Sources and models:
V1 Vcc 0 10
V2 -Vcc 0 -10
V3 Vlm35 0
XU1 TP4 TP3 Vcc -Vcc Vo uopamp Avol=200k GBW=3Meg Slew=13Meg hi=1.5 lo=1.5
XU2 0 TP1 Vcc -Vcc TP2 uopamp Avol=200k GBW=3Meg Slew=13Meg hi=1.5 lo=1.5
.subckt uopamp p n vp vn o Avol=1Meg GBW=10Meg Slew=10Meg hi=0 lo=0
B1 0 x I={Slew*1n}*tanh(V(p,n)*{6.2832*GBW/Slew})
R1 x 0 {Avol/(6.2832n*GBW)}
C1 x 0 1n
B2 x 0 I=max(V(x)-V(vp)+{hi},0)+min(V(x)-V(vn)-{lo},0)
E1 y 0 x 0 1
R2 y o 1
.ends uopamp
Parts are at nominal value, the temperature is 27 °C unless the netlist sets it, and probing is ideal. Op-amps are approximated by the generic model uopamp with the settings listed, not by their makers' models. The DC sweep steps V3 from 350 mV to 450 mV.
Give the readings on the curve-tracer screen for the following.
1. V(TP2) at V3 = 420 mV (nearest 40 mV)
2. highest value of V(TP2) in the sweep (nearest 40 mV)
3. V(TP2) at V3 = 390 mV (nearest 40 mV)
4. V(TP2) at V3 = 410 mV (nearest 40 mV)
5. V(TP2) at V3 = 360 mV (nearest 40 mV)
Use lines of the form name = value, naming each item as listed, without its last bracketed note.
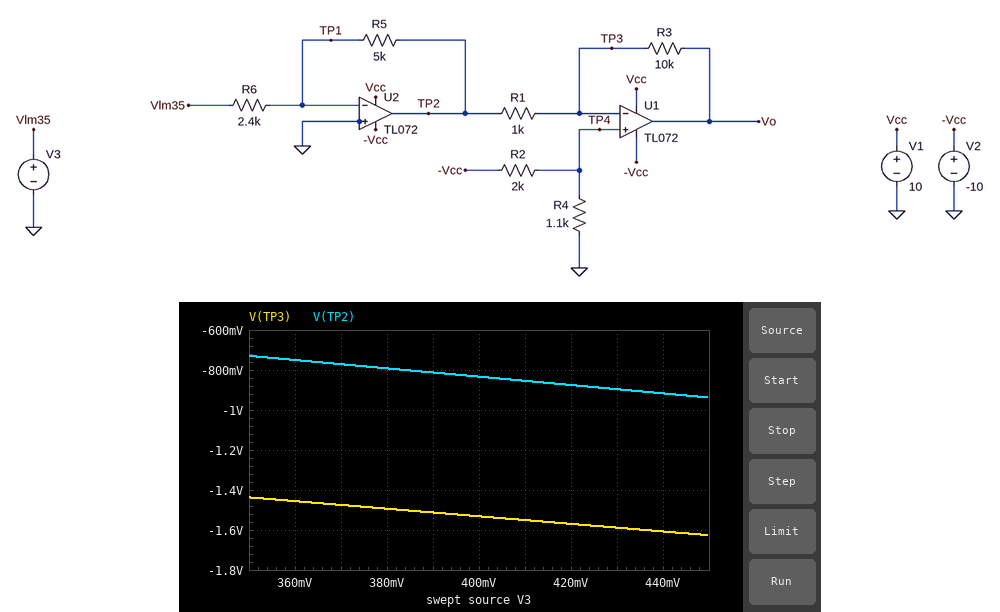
V(TP2) at V3 = 420 mV = -880 mV
highest value of V(TP2) in the sweep = -720 mV
V(TP2) at V3 = 390 mV = -800 mV
V(TP2) at V3 = 410 mV = -840 mV
V(TP2) at V3 = 360 mV = -760 mV
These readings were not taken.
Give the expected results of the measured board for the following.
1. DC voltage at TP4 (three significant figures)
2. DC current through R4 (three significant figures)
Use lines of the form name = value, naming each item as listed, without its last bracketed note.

DC voltage at TP4 = -3.55 V
DC current through R4 = 3.23 mA
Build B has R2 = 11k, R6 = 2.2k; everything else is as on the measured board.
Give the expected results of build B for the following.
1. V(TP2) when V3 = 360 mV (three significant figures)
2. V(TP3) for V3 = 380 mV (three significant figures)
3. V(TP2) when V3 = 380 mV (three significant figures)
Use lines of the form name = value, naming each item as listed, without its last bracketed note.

V(TP2) when V3 = 360 mV = -818 mV
V(TP3) for V3 = 380 mV = -909 mV
V(TP2) when V3 = 380 mV = -864 mV
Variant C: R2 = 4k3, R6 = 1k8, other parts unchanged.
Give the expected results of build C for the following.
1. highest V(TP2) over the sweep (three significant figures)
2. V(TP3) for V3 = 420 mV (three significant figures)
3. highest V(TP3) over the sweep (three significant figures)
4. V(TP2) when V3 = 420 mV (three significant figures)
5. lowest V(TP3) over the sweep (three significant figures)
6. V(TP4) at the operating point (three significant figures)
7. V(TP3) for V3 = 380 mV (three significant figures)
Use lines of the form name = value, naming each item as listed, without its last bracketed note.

highest V(TP2) over the sweep = -972 mV
V(TP3) for V3 = 420 mV = -1.83 V
highest V(TP3) over the sweep = -1.66 V
V(TP2) when V3 = 420 mV = -1.17 V
lowest V(TP3) over the sweep = -1.91 V
V(TP4) at the operating point = -2.04 V
V(TP3) for V3 = 380 mV = -1.73 V
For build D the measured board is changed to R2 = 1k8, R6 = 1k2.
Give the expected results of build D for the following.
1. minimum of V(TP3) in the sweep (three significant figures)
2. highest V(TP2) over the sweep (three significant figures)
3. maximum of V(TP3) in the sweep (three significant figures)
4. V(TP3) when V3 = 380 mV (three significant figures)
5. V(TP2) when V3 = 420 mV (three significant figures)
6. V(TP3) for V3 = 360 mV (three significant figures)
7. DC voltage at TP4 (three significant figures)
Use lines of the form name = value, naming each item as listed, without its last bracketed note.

minimum of V(TP3) in the sweep = -2.48 V
highest V(TP2) over the sweep = -1.46 V
maximum of V(TP3) in the sweep = -2.10 V
V(TP3) when V3 = 380 mV = -2.21 V
V(TP2) when V3 = 420 mV = -1.75 V
V(TP3) for V3 = 360 mV = -2.14 V
DC voltage at TP4 = -3.79 V
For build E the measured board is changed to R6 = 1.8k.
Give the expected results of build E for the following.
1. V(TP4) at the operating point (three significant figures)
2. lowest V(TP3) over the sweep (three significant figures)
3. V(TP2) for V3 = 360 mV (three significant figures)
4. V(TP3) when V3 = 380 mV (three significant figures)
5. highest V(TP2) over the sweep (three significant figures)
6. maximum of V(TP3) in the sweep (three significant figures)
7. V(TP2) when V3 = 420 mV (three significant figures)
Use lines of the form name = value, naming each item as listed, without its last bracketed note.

V(TP4) at the operating point = -3.55 V
lowest V(TP3) over the sweep = -1.91 V
V(TP2) for V3 = 360 mV = -1.00 V
V(TP3) when V3 = 380 mV = -1.73 V
highest V(TP2) over the sweep = -972 mV
maximum of V(TP3) in the sweep = -1.66 V
V(TP2) when V3 = 420 mV = -1.17 V
